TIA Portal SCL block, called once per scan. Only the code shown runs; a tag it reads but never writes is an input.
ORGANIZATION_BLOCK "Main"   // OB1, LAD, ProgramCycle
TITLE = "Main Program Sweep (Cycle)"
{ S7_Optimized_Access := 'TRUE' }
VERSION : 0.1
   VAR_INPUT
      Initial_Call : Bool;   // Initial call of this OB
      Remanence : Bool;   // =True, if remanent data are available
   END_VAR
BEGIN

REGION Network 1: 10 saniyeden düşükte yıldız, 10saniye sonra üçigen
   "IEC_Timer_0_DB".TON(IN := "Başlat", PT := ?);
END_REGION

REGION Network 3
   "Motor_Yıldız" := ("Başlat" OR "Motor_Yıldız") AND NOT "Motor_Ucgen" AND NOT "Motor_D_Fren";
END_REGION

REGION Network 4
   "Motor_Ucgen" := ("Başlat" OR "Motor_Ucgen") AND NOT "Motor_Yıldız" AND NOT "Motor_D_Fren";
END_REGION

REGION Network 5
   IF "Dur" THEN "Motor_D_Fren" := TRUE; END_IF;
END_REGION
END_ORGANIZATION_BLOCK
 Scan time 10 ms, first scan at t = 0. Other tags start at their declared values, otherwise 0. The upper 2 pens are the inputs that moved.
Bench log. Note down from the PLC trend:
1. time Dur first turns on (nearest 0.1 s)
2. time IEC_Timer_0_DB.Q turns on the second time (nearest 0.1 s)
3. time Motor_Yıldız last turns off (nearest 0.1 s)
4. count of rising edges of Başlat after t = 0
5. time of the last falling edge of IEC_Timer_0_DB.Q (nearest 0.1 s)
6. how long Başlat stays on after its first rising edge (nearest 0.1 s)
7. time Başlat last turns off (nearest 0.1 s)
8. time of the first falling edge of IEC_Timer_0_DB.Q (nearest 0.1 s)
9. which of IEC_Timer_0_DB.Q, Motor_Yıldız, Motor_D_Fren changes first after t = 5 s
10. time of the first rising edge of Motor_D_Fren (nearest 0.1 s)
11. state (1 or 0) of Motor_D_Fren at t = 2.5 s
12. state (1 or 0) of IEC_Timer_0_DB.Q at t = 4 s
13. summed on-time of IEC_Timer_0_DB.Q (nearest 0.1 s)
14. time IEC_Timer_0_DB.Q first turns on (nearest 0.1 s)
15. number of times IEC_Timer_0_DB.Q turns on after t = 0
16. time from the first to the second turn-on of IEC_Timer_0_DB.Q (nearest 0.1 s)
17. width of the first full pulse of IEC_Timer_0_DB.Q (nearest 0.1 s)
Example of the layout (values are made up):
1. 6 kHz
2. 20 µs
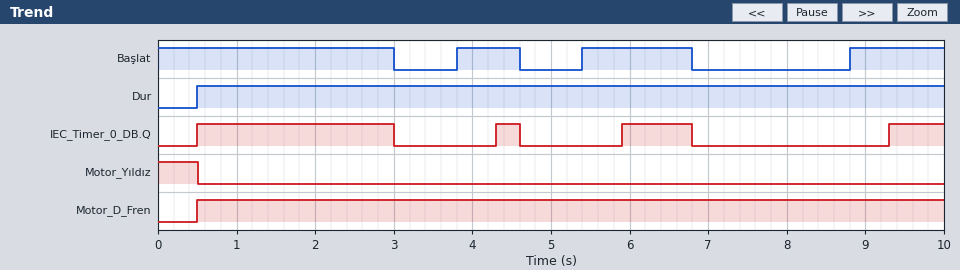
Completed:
1. 0.5 s
2. 4.3 s
3. 0.5 s
4. 3
5. 6.8 s
6. 0.8 s
7. 6.8 s
8. 3.0 s
9. IEC_Timer_0_DB.Q
10. 0.5 s
11. 1
12. 0
13. 4.4 s
14. 0.5 s
15. 4
16. 3.8 s
17. 2.5 s
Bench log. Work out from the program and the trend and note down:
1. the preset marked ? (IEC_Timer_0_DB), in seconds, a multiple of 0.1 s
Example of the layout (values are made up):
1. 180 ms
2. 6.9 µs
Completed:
1. 0.5 s
